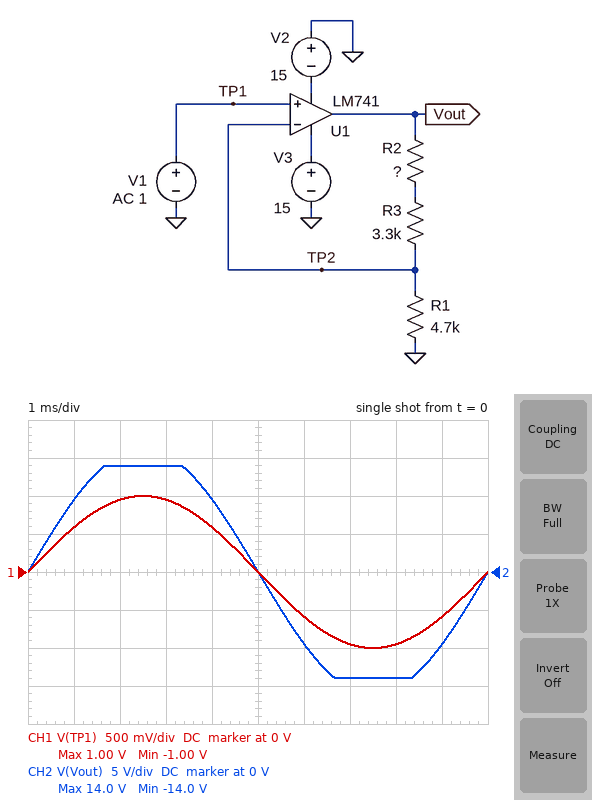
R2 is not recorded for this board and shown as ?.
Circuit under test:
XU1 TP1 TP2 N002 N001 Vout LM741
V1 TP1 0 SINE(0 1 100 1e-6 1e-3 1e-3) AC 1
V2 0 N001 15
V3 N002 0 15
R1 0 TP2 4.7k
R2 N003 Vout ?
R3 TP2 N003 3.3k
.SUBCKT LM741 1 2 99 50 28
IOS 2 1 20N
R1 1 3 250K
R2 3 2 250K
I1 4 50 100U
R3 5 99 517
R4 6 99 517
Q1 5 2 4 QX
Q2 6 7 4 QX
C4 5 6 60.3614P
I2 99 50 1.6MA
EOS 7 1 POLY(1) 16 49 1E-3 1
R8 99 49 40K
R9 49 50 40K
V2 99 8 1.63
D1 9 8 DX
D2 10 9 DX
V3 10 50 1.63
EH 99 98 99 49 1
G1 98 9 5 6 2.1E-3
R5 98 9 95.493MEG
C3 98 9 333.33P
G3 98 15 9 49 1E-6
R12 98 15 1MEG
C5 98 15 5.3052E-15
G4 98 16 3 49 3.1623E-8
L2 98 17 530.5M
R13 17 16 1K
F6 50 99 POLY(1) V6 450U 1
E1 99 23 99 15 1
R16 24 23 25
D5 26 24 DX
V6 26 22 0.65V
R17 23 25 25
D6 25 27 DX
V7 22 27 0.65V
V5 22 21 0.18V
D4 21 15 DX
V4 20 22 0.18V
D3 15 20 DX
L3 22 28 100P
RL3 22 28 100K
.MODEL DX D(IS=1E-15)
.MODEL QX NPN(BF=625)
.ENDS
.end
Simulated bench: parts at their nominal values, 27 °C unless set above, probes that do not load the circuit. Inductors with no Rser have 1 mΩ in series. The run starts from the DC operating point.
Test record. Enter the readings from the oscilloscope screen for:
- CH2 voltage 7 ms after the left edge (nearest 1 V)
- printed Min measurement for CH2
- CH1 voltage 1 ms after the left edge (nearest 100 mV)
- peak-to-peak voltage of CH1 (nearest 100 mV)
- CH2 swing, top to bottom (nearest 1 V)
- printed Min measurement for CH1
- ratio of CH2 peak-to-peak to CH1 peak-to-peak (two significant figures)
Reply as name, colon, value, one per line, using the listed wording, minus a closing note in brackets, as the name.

CH2 voltage 7 ms after the left edge: -14 V
printed Min measurement for CH2: -14.0 V
CH1 voltage 1 ms after the left edge: 600 mV
peak-to-peak voltage of CH1: 2.0 V
CH2 swing, top to bottom: 28 V
printed Min measurement for CH1: -1.00 V
ratio of CH2 peak-to-peak to CH1 peak-to-peak: 14
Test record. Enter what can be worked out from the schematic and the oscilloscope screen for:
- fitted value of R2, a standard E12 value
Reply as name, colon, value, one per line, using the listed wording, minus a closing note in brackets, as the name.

fitted value of R2, a standard E12 value: 68 kΩ
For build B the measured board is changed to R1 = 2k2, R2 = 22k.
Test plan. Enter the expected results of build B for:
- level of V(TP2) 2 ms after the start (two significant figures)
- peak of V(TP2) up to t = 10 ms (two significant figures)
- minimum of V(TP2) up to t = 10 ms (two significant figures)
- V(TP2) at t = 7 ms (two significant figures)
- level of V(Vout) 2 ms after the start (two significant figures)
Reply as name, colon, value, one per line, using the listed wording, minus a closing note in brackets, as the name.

level of V(TP2) 2 ms after the start: 950 mV
peak of V(TP2) up to t = 10 ms: 1.0 V
minimum of V(TP2) up to t = 10 ms: -1.0 V
V(TP2) at t = 7 ms: -950 mV
level of V(Vout) 2 ms after the start: 12 V
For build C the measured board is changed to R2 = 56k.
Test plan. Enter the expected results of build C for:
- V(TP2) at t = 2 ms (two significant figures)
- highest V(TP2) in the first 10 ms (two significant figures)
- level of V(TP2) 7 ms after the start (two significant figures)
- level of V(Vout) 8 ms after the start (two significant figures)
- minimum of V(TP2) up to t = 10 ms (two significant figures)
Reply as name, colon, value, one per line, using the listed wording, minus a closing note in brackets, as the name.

V(TP2) at t = 2 ms: 950 mV
highest V(TP2) in the first 10 ms: 1.0 V
level of V(TP2) 7 ms after the start: -950 mV
level of V(Vout) 8 ms after the start: -13 V
minimum of V(TP2) up to t = 10 ms: -1.0 V
